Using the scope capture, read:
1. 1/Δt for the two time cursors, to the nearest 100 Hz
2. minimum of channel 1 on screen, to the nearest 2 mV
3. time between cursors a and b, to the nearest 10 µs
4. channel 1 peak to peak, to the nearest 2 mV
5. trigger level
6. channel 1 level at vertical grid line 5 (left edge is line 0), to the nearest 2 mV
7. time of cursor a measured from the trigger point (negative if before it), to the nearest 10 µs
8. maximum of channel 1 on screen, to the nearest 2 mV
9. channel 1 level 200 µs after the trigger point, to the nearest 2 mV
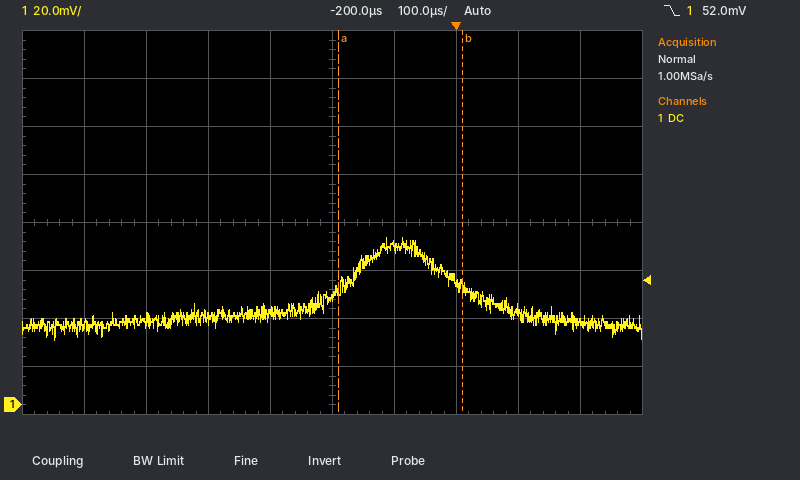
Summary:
5.0 kHz
28 mV
200 µs
42 mV
52.0 mV
46 mV
-190 µs
70 mV
34 mV
